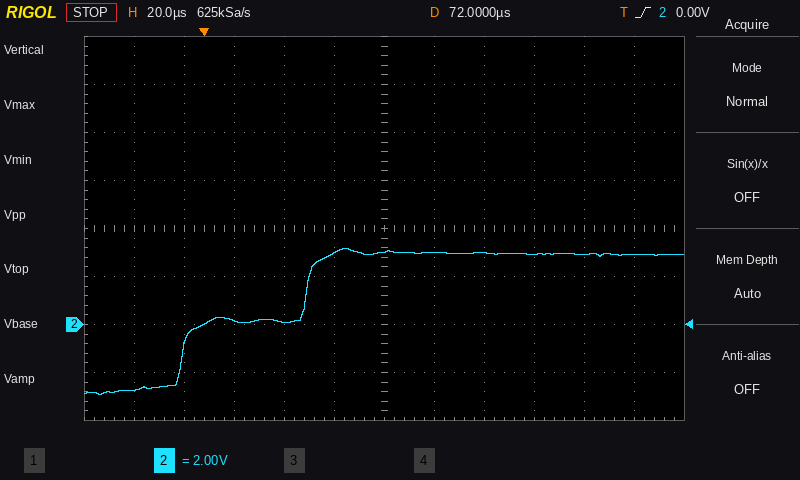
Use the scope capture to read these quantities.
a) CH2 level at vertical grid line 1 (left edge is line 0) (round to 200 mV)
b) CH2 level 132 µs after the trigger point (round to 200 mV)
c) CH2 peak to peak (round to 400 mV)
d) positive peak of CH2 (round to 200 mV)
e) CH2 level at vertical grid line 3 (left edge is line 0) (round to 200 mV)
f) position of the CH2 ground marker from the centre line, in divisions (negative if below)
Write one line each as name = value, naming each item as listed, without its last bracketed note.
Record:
CH2 level at vertical grid line 1 (left edge is line 0) = -2.8 V
CH2 level 132 µs after the trigger point = 3.0 V
CH2 peak to peak = 6.0 V
positive peak of CH2 = 3.2 V
CH2 level at vertical grid line 3 (left edge is line 0) = 200 mV
position of the CH2 ground marker from the centre line, in divisions = -2.0 div
